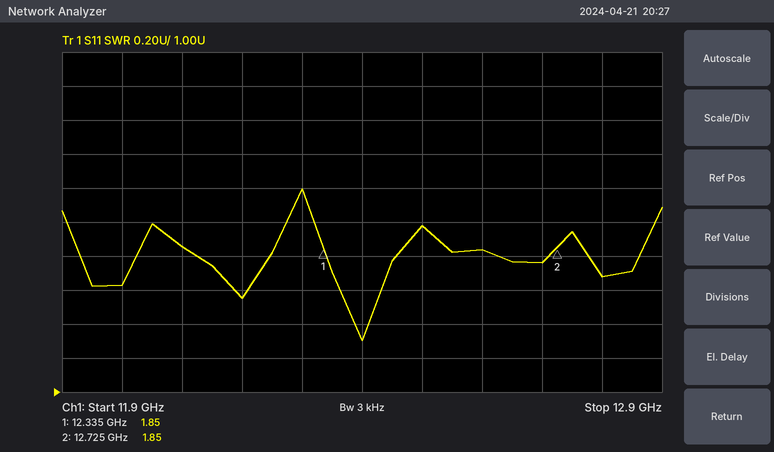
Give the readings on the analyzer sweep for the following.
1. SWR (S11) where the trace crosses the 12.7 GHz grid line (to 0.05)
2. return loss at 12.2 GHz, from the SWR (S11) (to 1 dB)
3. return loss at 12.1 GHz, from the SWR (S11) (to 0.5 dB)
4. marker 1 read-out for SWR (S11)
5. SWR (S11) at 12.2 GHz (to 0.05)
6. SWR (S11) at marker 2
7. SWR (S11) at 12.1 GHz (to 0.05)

1.75
13 dB
10.5 dB
1.85
1.55
1.85
1.85
